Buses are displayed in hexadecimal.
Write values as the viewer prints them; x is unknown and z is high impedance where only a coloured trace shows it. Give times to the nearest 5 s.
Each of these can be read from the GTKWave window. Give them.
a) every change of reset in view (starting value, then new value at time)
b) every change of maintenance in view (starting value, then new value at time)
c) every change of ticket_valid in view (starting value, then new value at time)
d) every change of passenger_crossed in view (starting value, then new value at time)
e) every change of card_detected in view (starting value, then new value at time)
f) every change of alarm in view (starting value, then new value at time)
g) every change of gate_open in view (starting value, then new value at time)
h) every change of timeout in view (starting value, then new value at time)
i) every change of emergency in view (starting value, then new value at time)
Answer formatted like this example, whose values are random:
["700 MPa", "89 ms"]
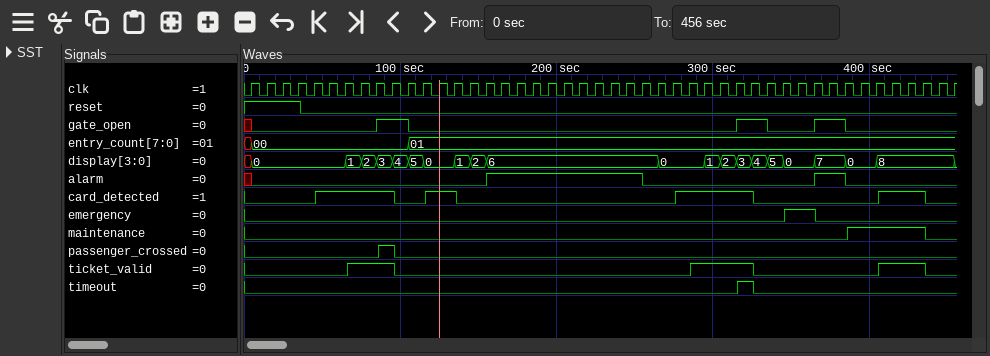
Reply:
["1, 0 at 35 s", "0, 1 at 385 s, 0 at 435 s", "0, 1 at 65 s, 0 at 95 s, 1 at 285 s, 0 at 325 s, 1 at 405 s, 0 at 435 s", "0, 1 at 85 s, 0 at 95 s", "0, 1 at 45 s, 0 at 95 s, 1 at 115 s, 0 at 135 s, 1 at 275 s, 0 at 325 s, 1 at 405 s, 0 at 435 s", "x, 0 at 5 s, 1 at 155 s, 0 at 255 s, 1 at 365 s, 0 at 385 s", "x, 0 at 5 s, 1 at 85 s, 0 at 105 s, 1 at 315 s, 0 at 335 s, 1 at 365 s, 0 at 385 s", "0, 1 at 315 s, 0 at 325 s", "0, 1 at 345 s, 0 at 365 s"]
